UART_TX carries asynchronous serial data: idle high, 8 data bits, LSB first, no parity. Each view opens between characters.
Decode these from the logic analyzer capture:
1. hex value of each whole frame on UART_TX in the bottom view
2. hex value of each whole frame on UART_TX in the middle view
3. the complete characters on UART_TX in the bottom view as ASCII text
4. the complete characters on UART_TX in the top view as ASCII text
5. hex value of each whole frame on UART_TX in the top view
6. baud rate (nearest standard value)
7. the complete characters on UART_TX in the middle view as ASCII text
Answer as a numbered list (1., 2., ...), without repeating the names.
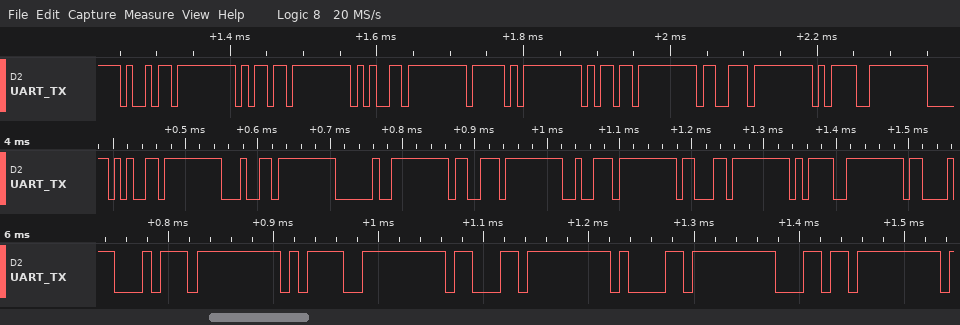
1. 74, 3D, 63, 61, 6C
2. 65, 64, 20, 73, 72, 63, 3D
3. "t=cal"
4. "ime_ms="
5. 69, 6D, 65, 5F, 6D, 73, 3D
6. 115200 baud
7. "ed src="
